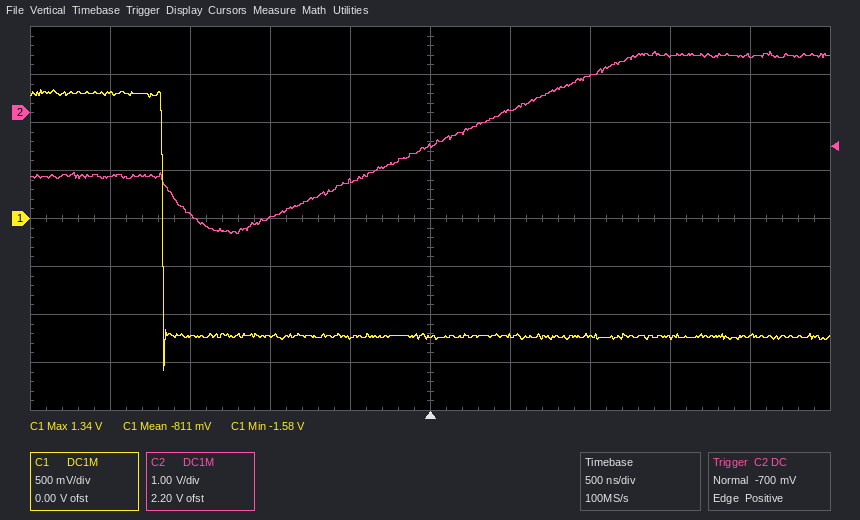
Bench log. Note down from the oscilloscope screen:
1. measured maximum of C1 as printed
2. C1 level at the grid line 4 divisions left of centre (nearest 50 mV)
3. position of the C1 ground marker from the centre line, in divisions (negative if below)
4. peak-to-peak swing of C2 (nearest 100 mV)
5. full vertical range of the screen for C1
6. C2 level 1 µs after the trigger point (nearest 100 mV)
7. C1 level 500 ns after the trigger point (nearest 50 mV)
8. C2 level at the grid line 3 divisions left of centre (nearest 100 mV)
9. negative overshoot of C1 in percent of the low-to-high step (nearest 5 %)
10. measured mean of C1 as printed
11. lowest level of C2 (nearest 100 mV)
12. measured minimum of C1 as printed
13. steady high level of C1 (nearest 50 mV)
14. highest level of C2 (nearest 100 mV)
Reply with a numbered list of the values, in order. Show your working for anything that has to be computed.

1. 1.34 V
2. 1.30 V
3. 0.0 div
4. 1.3 V − (-2.5 V) = 3.8 V
5. 4 V
6. 800 mV
7. -1.20 V
8. -2.1 V
9. 15 %
10. -811 mV
11. -2.5 V
12. -1.58 V
13. 1.30 V
14. 1.3 V
